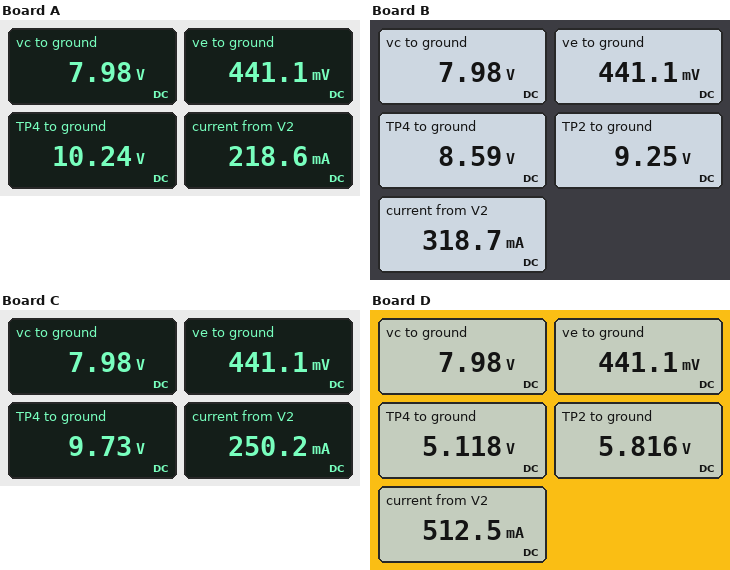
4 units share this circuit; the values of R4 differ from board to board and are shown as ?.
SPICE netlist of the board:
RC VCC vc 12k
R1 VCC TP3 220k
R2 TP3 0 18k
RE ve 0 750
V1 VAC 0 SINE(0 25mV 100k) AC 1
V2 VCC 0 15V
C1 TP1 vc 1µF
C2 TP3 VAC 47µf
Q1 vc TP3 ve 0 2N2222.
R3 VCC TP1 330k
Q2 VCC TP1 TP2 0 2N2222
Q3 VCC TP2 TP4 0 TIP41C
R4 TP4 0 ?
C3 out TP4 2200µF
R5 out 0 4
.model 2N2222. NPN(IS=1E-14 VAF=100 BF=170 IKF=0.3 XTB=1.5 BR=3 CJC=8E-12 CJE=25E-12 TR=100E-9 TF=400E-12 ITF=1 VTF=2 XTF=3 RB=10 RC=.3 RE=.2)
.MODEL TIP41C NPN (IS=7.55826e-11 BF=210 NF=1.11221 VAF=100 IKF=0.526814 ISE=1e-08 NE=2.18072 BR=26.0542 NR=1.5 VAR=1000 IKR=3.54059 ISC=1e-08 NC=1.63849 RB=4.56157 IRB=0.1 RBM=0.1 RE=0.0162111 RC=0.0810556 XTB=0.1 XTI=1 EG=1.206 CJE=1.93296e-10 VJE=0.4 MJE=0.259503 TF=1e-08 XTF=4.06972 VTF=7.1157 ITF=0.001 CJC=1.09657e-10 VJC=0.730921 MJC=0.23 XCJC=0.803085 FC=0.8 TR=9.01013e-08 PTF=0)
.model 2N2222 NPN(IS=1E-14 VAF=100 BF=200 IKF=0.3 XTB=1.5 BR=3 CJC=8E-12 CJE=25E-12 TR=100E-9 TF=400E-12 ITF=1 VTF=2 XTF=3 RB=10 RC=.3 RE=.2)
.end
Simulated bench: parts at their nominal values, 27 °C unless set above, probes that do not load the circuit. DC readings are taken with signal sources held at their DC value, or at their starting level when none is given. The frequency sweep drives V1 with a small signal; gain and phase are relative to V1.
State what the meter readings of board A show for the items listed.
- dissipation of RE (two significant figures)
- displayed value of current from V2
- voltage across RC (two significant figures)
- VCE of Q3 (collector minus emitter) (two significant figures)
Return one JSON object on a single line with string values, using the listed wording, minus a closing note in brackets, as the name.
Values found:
{"dissipation of RE": "260 µW", "displayed value of current from V2": "218.6 mA", "voltage across RC": "7.0 V", "VCE of Q3 (collector minus emitter)": "4.8 V"}
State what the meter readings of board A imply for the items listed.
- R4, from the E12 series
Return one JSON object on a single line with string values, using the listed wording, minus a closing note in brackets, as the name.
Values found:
{"R4, from the E12 series": "47 Ω"}
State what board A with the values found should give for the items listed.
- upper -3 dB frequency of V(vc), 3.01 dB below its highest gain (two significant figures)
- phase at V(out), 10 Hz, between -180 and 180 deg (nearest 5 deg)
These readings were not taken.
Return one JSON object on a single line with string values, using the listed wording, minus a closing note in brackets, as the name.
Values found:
{"upper -3 dB frequency of V(vc), 3.01 dB below its highest gain": "210 kHz", "phase at V(out), 10 Hz, between -180 and 180 deg": "-115 deg"}
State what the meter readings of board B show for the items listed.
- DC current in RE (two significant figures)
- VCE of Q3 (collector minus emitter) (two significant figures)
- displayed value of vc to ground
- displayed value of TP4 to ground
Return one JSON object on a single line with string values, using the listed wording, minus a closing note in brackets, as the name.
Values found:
{"DC current in RE": "590 µA", "VCE of Q3 (collector minus emitter)": "6.4 V", "displayed value of vc to ground": "7.98 V", "displayed value of TP4 to ground": "8.59 V"}
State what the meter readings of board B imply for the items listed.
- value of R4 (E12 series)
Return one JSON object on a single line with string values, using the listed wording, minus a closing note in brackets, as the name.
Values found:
{"value of R4": "27 Ω"}
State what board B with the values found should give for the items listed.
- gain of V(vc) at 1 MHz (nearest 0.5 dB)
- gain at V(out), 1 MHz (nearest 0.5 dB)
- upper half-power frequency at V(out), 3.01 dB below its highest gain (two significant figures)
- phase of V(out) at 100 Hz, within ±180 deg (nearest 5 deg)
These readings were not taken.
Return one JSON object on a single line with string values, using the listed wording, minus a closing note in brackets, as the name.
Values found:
{"gain of V(vc) at 1 MHz": "11.0 dB", "gain at V(out), 1 MHz": "7.5 dB", "upper half-power frequency at V(out), 3.01 dB below its highest gain": "280 kHz", "phase of V(out) at 100 Hz, within ±180 deg": "-170 deg"}
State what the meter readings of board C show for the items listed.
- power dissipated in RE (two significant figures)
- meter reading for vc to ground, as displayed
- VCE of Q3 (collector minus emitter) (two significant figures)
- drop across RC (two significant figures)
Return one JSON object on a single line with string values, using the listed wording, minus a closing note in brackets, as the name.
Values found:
{"power dissipated in RE": "260 µW", "meter reading for vc to ground, as displayed": "7.98 V", "VCE of Q3 (collector minus emitter)": "5.3 V", "drop across RC": "7.0 V"}
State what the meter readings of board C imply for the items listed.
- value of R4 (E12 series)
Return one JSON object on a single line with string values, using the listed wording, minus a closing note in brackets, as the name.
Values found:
{"value of R4": "39 Ω"}
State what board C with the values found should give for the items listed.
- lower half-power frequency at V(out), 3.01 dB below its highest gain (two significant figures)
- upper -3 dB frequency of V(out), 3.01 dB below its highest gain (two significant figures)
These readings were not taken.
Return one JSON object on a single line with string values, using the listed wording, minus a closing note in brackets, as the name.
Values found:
{"lower half-power frequency at V(out), 3.01 dB below its highest gain": "16 Hz", "upper -3 dB frequency of V(out), 3.01 dB below its highest gain": "260 kHz"}
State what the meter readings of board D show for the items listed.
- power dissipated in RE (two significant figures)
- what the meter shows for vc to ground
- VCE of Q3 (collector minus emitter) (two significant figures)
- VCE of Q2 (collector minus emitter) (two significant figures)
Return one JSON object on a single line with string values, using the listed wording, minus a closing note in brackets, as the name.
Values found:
{"power dissipated in RE": "260 µW", "what the meter shows for vc to ground": "7.98 V", "VCE of Q3 (collector minus emitter)": "9.9 V", "VCE of Q2 (collector minus emitter)": "9.2 V"}
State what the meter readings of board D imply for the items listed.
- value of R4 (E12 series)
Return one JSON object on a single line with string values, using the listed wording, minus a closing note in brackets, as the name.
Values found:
{"value of R4": "10 Ω"}
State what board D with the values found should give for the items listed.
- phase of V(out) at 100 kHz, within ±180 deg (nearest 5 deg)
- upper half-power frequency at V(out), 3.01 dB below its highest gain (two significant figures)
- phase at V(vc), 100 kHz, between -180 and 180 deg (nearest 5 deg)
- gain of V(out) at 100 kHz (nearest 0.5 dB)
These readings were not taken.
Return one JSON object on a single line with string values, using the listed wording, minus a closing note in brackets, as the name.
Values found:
{"phase of V(out) at 100 kHz, within ±180 deg": "160 deg", "upper half-power frequency at V(out), 3.01 dB below its highest gain": "320 kHz", "phase at V(vc), 100 kHz, between -180 and 180 deg": "165 deg", "gain of V(out) at 100 kHz": "20.0 dB"}
